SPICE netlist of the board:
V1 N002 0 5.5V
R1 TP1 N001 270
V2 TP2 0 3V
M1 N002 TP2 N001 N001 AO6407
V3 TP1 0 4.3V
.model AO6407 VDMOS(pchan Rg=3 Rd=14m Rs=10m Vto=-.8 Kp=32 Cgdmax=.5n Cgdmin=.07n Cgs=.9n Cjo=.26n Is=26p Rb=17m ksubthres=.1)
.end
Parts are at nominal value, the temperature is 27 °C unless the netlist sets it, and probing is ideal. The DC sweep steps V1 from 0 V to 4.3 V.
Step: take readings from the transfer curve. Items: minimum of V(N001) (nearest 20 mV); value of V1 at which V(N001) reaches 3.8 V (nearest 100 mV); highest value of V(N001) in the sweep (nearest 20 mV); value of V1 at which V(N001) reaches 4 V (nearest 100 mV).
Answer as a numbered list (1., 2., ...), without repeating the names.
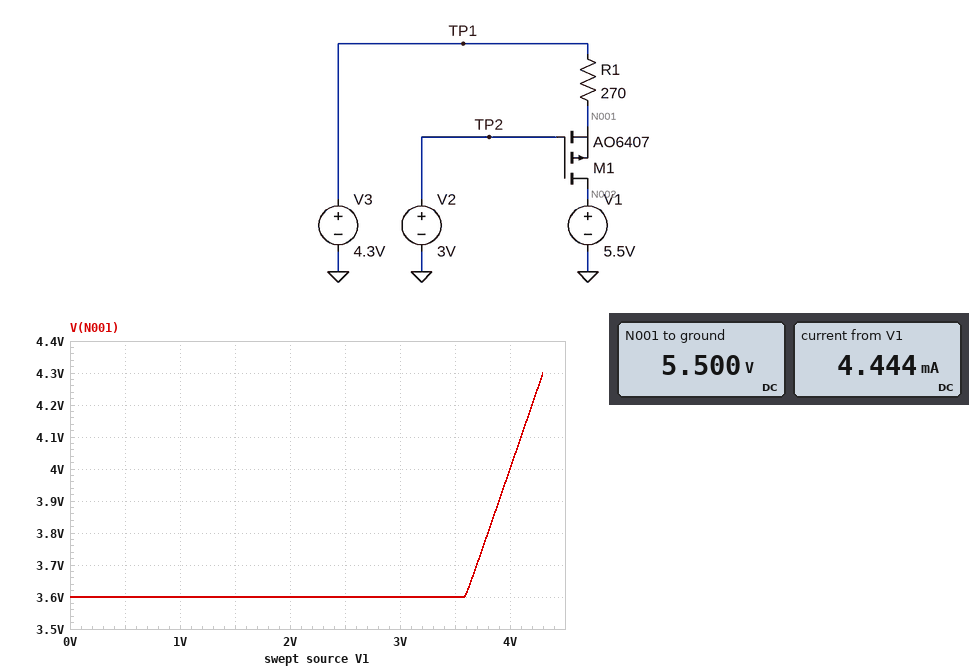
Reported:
1. 3.60 V
2. 3.8 V
3. 4.30 V
4. 4.0 V
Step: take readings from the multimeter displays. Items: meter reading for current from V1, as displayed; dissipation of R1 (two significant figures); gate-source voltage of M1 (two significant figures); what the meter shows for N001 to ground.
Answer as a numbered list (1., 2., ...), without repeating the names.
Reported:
1. 4.444 mA
2. 5.3 mW
3. -2.5 V
4. 5.500 V
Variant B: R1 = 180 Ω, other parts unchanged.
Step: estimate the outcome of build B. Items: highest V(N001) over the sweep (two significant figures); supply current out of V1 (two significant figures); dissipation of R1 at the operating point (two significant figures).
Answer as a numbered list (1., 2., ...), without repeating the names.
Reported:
1. 4.3 V
2. 6.7 mA
3. 8.0 mW
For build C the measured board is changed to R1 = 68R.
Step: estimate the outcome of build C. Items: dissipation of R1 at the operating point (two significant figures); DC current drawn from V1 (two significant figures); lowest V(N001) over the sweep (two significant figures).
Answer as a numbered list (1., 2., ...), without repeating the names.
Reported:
1. 21 mW
2. 18 mA
3. 3.7 V
